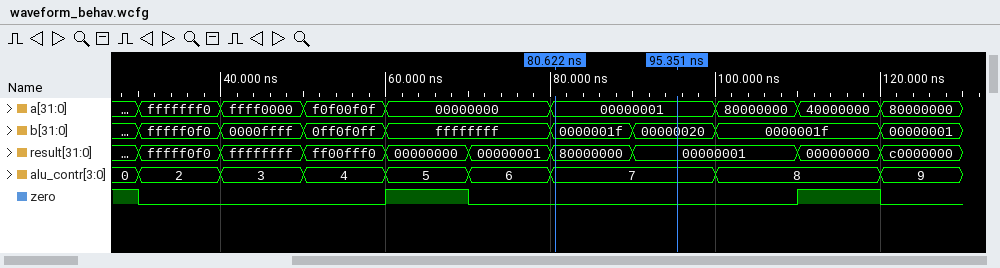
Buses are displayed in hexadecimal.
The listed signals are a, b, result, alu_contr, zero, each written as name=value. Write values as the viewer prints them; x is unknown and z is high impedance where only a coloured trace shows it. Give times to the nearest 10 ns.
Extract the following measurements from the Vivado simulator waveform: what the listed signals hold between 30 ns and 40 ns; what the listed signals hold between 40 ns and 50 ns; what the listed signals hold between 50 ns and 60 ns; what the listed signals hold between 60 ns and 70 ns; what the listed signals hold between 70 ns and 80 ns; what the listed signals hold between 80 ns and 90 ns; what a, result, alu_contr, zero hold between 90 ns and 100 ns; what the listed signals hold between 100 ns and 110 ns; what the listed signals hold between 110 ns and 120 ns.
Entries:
a=fffffff0, b=fffff0f0, result=fffff0f0, alu_contr=2, zero=0
a=ffff0000, b=0000ffff, result=ffffffff, alu_contr=3, zero=0
a=f0f00f0f, b=0ff0f0ff, result=ff00fff0, alu_contr=4, zero=0
a=00000000, b=ffffffff, result=00000000, alu_contr=5, zero=1
a=00000000, b=ffffffff, result=00000001, alu_contr=6, zero=0
a=00000001, b=0000001f, result=80000000, alu_contr=7, zero=0
a=00000001, result=00000001, alu_contr=7, zero=0
a=80000000, b=0000001f, result=00000001, alu_contr=8, zero=0
a=40000000, b=0000001f, result=00000000, alu_contr=8, zero=1
